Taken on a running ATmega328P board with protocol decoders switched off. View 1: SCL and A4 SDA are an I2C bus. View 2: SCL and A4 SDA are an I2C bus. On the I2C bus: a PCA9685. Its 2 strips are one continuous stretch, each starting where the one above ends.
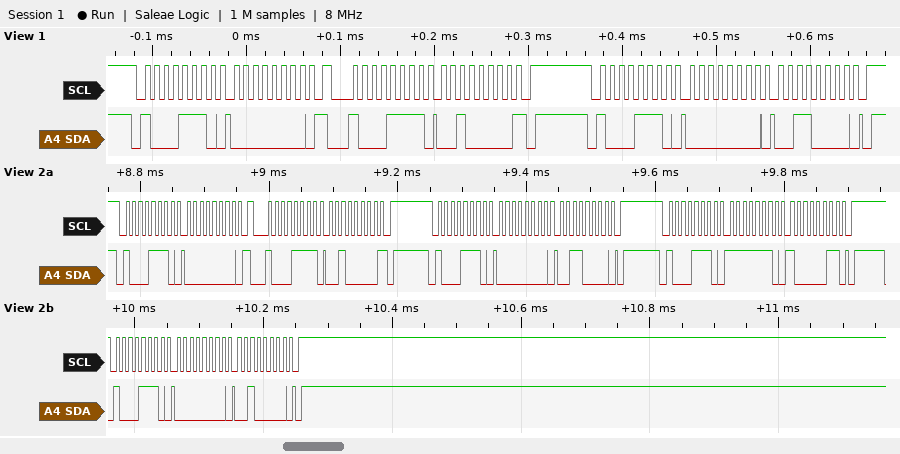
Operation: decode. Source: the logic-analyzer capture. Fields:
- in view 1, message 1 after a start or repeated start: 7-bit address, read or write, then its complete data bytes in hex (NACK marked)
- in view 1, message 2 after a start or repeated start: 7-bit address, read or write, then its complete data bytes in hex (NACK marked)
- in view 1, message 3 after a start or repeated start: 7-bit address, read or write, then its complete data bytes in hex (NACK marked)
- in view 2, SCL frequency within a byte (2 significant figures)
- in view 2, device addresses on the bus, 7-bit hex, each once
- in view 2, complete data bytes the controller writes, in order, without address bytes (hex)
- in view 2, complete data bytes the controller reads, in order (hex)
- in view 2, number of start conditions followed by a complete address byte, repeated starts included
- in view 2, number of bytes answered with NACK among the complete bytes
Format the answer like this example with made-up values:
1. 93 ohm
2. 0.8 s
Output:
1. 0x47 write: 00
2. 0x47 read: 20 NACK
3. 0x47 write: 00 30
4. 100 kHz
5. 0x47
6. 00 00 30 FE 83 00 20
7. 20
8. 5
9. 1
